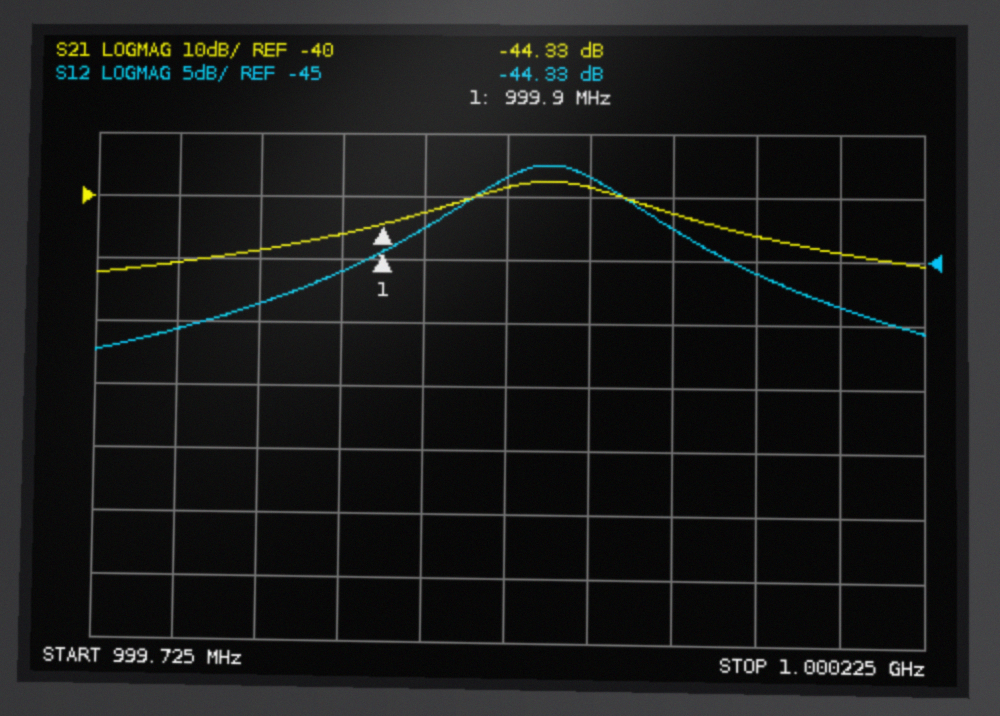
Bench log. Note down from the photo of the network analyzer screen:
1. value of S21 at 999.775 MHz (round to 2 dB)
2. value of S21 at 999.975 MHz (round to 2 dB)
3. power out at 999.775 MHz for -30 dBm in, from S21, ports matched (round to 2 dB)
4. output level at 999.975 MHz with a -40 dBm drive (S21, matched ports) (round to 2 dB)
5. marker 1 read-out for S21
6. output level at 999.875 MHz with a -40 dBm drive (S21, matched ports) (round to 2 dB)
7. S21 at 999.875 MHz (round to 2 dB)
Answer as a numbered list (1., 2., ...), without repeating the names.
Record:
1. -50 dB
2. -38 dB
3. -80 dBm
4. -78 dBm
5. -44.33 dB
6. -86 dBm
7. -46 dB
